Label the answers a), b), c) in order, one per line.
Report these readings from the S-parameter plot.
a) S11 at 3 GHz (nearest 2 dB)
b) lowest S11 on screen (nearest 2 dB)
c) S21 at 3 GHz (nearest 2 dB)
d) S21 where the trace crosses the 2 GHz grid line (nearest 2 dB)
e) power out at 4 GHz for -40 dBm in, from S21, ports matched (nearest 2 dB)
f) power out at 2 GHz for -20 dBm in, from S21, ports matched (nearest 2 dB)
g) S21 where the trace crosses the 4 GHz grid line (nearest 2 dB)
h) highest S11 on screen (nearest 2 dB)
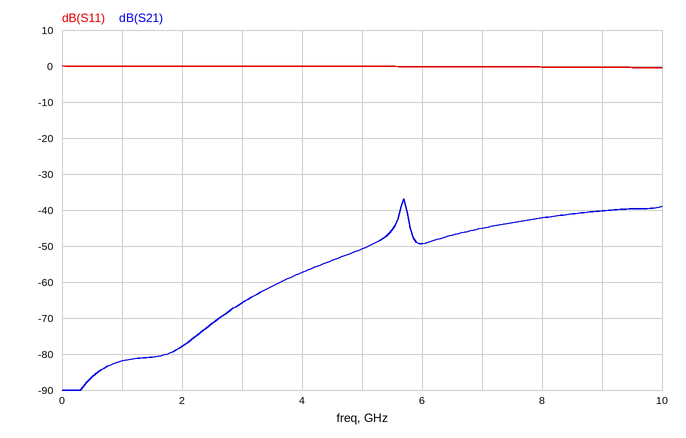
a) 0 dB
b) 0 dB
c) -66 dB
d) -78 dB
e) -98 dBm
f) -98 dBm
g) -58 dB
h) 0 dB
